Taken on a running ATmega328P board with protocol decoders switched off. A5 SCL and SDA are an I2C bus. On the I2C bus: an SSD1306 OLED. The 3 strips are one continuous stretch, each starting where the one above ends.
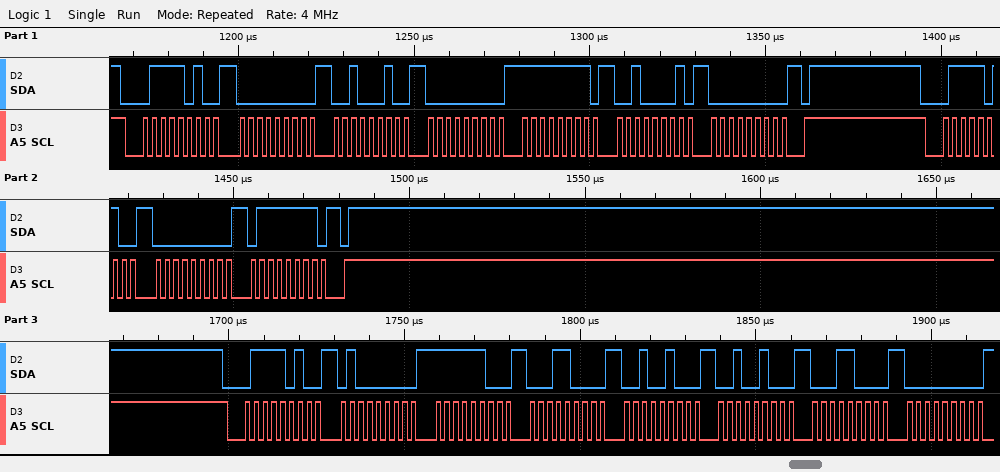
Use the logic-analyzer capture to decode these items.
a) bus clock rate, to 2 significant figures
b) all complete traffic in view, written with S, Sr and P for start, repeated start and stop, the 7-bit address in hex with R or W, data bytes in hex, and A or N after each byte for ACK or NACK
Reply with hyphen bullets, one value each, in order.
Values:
- 400 kHz
- S 3DW A 00 A 22 A 00 A FF A 21 A 00 A P S 3DW A 00 A 7F A P S 3DW A 40 A FC A 18 A 24 A 24 A 18 A 00 A
